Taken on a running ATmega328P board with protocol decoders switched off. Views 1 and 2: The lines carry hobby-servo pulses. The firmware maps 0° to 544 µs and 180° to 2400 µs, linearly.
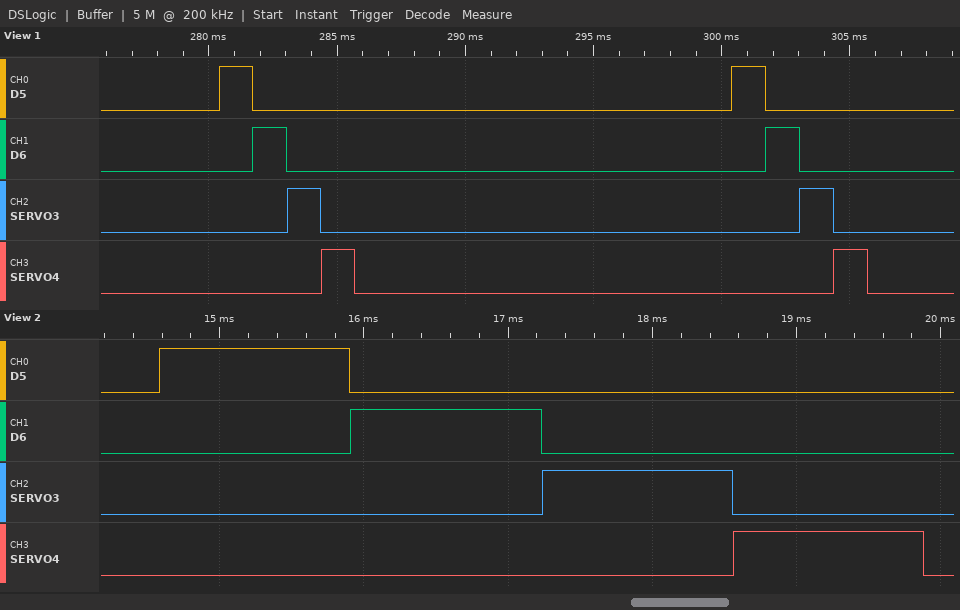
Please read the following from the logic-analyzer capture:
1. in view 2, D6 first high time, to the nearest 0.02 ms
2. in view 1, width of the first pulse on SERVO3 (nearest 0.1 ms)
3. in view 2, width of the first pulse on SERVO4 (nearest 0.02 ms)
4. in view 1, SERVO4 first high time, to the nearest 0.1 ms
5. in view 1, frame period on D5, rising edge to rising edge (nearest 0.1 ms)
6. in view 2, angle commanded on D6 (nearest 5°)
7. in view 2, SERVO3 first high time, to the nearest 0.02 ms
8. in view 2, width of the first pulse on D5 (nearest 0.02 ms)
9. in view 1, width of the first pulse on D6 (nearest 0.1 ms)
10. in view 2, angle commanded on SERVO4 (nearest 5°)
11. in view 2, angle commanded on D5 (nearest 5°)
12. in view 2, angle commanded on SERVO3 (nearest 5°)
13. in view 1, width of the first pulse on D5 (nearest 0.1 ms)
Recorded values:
1.32 ms
1.3 ms
1.32 ms
1.3 ms
20.0 ms
75°
1.32 ms
1.32 ms
1.3 ms
75°
75°
75°
1.3 ms
